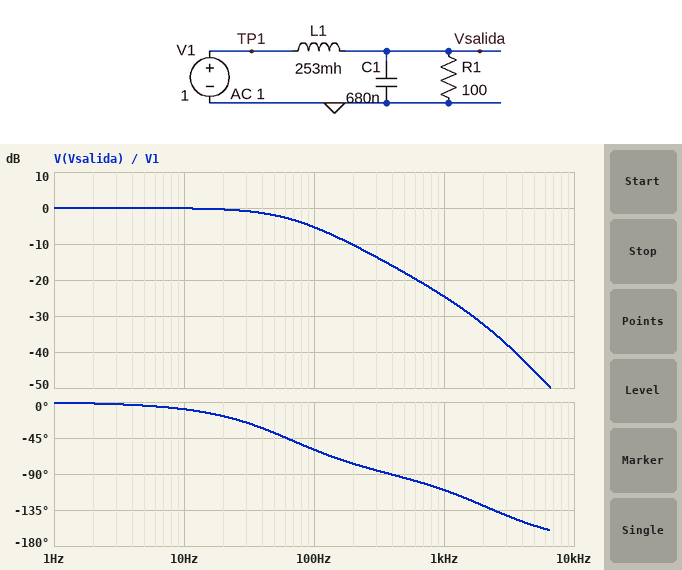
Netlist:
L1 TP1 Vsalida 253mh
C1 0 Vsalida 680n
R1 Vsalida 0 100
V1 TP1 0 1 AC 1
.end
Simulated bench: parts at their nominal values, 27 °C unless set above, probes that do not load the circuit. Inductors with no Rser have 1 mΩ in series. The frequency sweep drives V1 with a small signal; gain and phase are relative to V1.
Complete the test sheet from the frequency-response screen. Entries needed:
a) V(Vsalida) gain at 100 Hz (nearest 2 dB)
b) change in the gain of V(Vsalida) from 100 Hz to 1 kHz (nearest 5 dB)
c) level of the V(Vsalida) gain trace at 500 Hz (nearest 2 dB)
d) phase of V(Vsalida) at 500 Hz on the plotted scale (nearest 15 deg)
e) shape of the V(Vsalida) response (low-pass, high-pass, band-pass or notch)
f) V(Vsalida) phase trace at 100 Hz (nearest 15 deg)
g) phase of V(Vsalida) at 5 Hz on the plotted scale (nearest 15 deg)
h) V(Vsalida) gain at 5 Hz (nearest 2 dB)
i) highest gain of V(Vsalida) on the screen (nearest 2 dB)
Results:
-6 dB
-20 dB
-18 dB
-90 deg
low-pass
-60 deg
0 deg
0 dB
0 dB
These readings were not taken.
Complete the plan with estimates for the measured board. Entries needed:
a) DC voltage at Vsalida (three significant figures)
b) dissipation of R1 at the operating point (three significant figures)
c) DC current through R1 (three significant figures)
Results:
1.00 V
10.0 mW
10.0 mA
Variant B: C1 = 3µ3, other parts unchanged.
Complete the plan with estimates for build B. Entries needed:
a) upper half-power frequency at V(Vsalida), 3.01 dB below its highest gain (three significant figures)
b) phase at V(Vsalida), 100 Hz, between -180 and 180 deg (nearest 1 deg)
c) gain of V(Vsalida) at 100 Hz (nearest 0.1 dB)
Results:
72.1 Hz
-67 deg
-4.7 dB
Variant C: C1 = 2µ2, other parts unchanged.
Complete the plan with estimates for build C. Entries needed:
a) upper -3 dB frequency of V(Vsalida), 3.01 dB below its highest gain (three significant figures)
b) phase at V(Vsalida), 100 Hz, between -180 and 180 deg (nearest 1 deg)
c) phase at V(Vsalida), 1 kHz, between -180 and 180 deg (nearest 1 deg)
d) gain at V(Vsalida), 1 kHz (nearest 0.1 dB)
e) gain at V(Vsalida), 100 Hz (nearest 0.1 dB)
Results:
68.8 Hz
-64 deg
-143 deg
-28.4 dB
-5.0 dB
